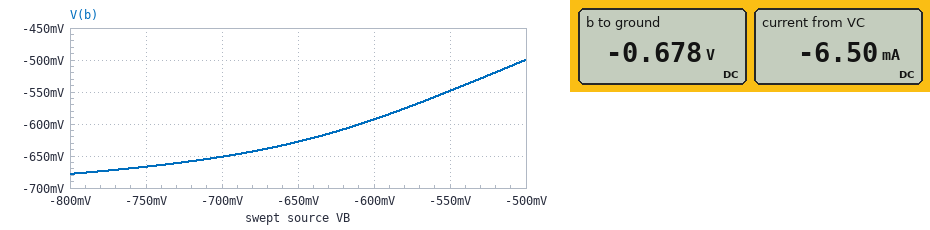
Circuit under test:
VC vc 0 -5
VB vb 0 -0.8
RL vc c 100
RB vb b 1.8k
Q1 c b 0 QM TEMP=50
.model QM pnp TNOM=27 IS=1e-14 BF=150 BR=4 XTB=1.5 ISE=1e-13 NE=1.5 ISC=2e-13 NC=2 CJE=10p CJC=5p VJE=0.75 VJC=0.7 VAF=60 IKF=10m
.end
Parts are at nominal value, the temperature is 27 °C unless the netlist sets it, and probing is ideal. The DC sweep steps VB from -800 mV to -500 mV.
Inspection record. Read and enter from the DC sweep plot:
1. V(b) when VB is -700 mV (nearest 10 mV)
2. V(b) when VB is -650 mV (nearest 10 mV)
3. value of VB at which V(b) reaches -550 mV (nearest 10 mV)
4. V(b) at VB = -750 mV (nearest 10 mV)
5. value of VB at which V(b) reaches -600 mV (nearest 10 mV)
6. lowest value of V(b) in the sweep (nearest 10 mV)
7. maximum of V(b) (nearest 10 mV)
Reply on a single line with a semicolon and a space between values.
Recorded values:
-650 mV; -630 mV; -550 mV; -670 mV; -610 mV; -680 mV; -500 mV
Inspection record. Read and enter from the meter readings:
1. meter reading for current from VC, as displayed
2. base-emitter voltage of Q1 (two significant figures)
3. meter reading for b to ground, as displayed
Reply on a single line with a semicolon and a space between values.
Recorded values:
-6.50 mA; -680 mV; -0.678 V
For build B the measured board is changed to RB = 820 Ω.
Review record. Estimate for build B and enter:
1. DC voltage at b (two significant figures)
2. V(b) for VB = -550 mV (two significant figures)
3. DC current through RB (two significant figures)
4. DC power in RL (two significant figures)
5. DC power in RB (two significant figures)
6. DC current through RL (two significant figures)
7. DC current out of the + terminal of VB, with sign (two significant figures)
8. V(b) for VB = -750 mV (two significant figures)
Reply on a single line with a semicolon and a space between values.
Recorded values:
-700 mV; -550 mV; 130 µA; 10 mW; 13 µW; 10 mA; -130 µA; -680 mV
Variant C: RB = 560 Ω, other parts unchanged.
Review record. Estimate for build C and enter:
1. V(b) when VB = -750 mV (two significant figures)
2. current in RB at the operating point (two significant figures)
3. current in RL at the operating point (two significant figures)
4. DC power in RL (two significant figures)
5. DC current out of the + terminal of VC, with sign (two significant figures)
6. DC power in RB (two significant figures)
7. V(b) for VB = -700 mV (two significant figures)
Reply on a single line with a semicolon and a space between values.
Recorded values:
-690 mV; 170 µA; 12 mA; 15 mW; -12 mA; 16 µW; -670 mV
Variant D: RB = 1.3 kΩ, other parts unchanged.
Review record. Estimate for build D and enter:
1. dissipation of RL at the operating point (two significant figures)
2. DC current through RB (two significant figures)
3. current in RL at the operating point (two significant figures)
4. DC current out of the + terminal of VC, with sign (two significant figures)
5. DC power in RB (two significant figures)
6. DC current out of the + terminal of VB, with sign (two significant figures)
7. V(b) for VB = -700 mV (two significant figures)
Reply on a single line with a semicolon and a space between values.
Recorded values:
6.2 mW; 88 µA; 7.9 mA; -7.9 mA; 10 µW; -88 µA; -660 mV
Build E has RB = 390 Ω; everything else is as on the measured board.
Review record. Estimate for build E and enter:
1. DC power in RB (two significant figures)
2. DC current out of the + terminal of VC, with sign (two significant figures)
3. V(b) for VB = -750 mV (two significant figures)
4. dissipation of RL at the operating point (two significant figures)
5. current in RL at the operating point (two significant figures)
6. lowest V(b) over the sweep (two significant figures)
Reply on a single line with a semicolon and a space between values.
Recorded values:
20 µW; -15 mA; -700 mV; 22 mW; 15 mA; -710 mV
